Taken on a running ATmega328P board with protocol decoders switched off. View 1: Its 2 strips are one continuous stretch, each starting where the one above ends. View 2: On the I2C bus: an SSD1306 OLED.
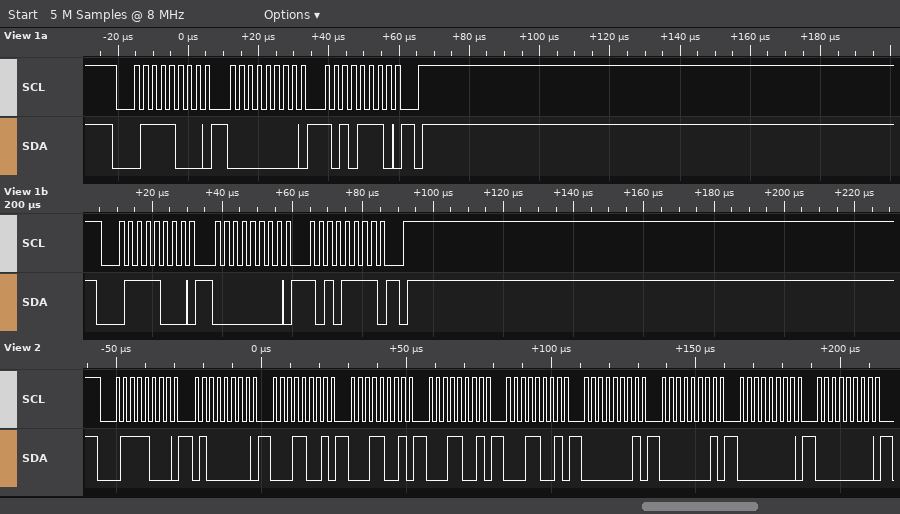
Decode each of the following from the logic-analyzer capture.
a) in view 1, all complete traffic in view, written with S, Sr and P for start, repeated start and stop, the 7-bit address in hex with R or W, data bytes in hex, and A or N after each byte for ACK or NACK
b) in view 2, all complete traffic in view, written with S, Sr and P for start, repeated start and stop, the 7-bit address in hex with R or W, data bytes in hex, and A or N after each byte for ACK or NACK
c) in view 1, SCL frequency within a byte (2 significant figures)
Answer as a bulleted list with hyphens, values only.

- S 3CW A 00 A AE A P S 3CW A 00 A AF A P
- S 3CW A 40 A 19 A 19 A 19 A 19 A 01 A 01 A 00 A 00 A
- 400 kHz
